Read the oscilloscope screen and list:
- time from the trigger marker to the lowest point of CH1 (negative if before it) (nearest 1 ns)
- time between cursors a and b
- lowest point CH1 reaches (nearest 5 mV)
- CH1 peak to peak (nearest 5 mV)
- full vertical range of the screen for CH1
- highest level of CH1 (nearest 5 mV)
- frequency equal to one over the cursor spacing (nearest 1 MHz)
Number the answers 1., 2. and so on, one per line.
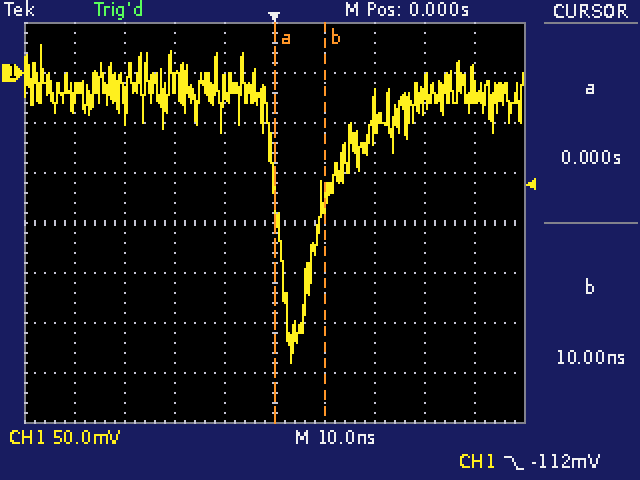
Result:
1. +3 ns
2. 10 ns
3. -290 mV
4. 320 mV
5. 400 mV
6. 30 mV
7. 100 MHz
